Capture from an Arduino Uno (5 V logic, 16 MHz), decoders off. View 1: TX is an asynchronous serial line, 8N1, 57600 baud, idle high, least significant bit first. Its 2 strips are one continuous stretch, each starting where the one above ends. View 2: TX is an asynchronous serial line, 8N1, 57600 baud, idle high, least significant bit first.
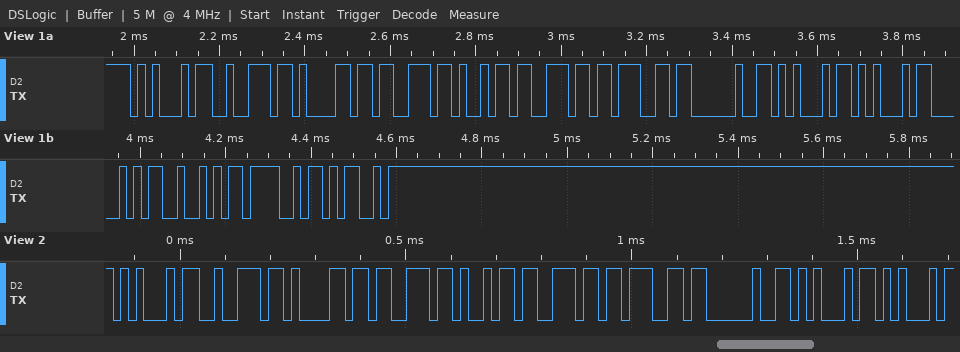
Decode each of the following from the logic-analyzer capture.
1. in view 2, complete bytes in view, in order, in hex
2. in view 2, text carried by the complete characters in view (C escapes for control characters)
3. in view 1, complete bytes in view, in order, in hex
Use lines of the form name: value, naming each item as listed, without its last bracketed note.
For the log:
in view 2, complete bytes in view, in order, in hex: 45 72 61 73 69 6E 67 20 45 45
in view 2, text carried by the complete characters in view: "Erasing EE"
in view 1, complete bytes in view, in order, in hex: 45 72 61 73 69 6E 67 20 45 45 50 52 4F 4D
